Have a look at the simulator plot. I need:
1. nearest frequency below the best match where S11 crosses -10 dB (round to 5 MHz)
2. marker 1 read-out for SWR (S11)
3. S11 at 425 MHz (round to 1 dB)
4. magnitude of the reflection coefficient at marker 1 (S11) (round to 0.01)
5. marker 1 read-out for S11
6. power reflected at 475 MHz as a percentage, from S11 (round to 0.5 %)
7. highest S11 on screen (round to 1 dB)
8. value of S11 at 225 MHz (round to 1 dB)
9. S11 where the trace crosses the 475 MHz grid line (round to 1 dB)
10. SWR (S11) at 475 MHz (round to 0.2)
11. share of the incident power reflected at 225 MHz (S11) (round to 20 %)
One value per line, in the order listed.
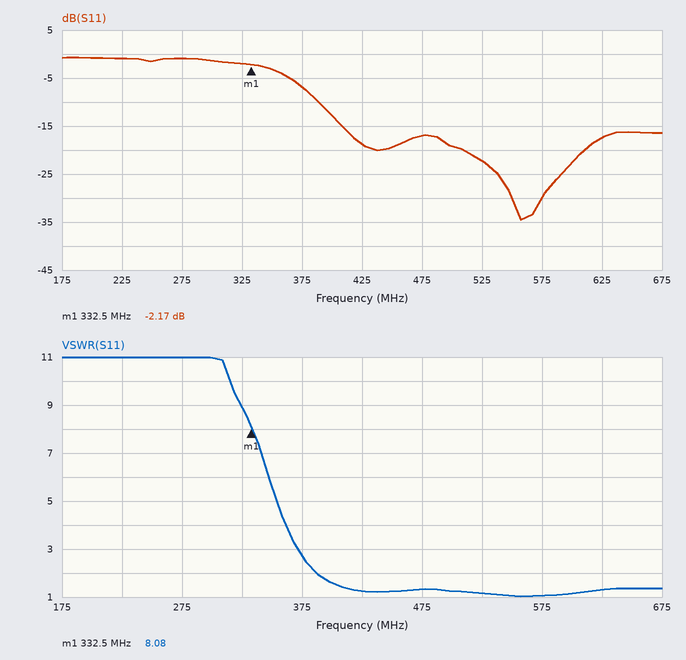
390 MHz
8.08
-19 dB
0.78
-2.17 dB
2.0 %
-1 dB
-1 dB
-17 dB
1.4
80 %
